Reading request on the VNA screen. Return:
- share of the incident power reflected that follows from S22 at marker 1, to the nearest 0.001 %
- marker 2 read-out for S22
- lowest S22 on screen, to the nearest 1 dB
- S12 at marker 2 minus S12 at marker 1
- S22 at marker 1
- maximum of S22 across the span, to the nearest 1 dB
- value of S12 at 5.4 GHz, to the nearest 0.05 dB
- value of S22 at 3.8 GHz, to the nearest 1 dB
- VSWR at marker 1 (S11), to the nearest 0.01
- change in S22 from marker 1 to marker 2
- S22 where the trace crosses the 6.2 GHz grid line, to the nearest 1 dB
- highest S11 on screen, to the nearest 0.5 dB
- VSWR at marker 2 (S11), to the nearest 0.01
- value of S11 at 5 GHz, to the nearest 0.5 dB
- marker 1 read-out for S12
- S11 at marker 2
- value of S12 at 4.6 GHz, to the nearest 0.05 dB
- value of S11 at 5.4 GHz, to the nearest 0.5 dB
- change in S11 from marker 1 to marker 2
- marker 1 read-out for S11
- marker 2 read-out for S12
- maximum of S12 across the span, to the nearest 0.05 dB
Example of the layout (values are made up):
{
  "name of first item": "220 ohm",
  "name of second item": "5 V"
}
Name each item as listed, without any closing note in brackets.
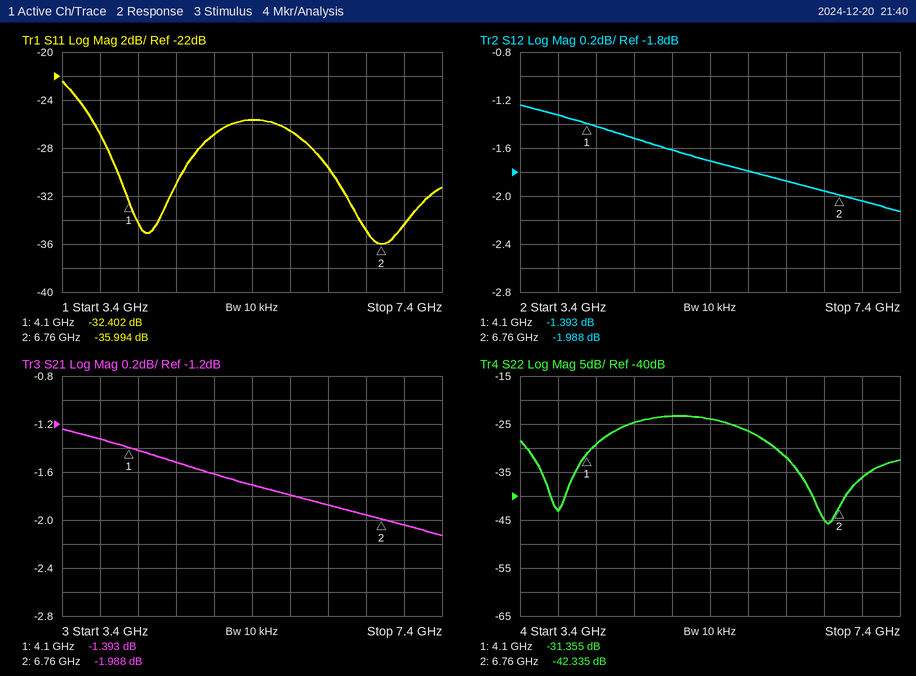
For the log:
{
  "share of the incident power reflected that follows from S22 at marker 1, to the nearest 0.001 %": "0.073 %",
  "marker 2 read-out for S22": "-42.335 dB",
  "lowest S22 on screen, to the nearest 1 dB": "-46 dB",
  "S12 at marker 2 minus S12 at marker 1": "-0.595 dB",
  "S22 at marker 1": "-31.355 dB",
  "maximum of S22 across the span, to the nearest 1 dB": "-23 dB",
  "value of S12 at 5.4 GHz, to the nearest 0.05 dB": "-1.70 dB",
  "value of S22 at 3.8 GHz, to the nearest 1 dB": "-43 dB",
  "VSWR at marker 1 (S11), to the nearest 0.01": "1.05",
  "change in S22 from marker 1 to marker 2": "-10.980 dB",
  "S22 where the trace crosses the 6.2 GHz grid line, to the nearest 1 dB": "-32 dB",
  "highest S11 on screen, to the nearest 0.5 dB": "-22.5 dB",
  "VSWR at marker 2 (S11), to the nearest 0.01": "1.03",
  "value of S11 at 5 GHz, to the nearest 0.5 dB": "-27.0 dB",
  "marker 1 read-out for S12": "-1.393 dB",
  "S11 at marker 2": "-35.994 dB",
  "value of S12 at 4.6 GHz, to the nearest 0.05 dB": "-1.50 dB",
  "value of S11 at 5.4 GHz, to the nearest 0.5 dB": "-25.5 dB",
  "change in S11 from marker 1 to marker 2": "-3.592 dB",
  "marker 1 read-out for S11": "-32.402 dB",
  "marker 2 read-out for S12": "-1.988 dB",
  "maximum of S12 across the span, to the nearest 0.05 dB": "-1.25 dB"
}
